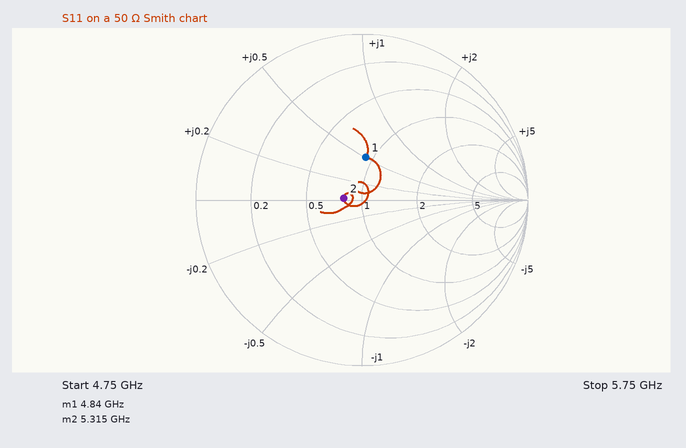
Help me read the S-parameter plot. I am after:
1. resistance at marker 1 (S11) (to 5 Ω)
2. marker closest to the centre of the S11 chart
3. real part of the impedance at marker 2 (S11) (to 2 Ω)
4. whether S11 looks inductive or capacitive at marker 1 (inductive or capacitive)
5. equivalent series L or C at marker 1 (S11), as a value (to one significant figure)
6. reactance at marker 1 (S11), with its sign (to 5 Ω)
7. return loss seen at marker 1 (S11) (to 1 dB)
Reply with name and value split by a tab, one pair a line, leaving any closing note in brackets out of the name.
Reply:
resistance at marker 1 (S11)	45 Ω
marker closest to the centre of the S11 chart	marker 2
real part of the impedance at marker 2 (S11)	40 Ω
whether S11 looks inductive or capacitive at marker 1	inductive
equivalent series L or C at marker 1 (S11), as a value	800 pH
reactance at marker 1 (S11), with its sign	+25 Ω
return loss seen at marker 1 (S11)	12 dB
